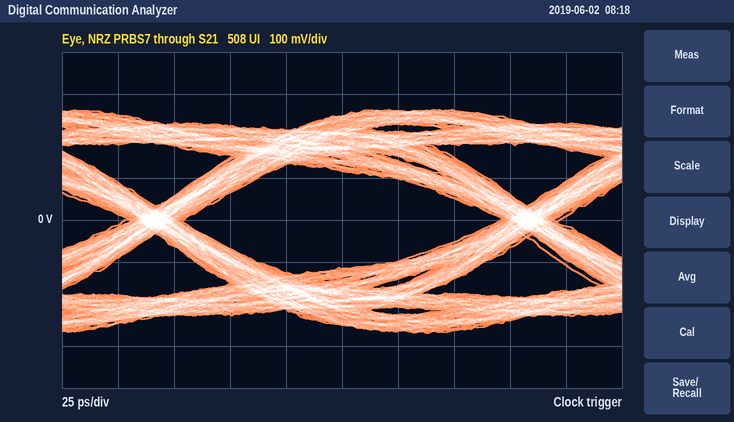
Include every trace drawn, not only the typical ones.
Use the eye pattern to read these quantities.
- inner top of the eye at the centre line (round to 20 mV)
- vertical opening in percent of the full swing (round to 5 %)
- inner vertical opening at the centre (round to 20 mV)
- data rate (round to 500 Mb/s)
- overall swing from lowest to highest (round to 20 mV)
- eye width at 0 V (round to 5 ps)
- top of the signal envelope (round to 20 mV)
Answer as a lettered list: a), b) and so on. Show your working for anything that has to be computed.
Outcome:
a) 120 mV
b) 240 mV / 540 mV ≈ 44.4 %, so 45 % to the nearest 5 %
c) 240 mV
d) 6.0 Gb/s
e) 540 mV
f) 140 ps
g) 260 mV
